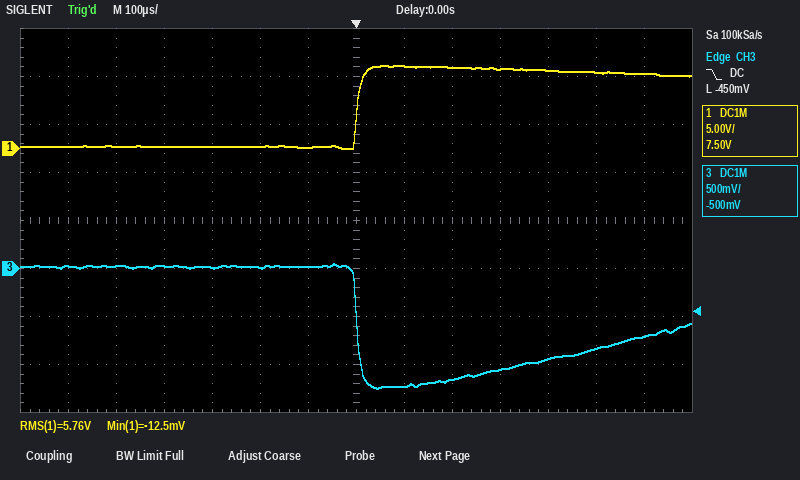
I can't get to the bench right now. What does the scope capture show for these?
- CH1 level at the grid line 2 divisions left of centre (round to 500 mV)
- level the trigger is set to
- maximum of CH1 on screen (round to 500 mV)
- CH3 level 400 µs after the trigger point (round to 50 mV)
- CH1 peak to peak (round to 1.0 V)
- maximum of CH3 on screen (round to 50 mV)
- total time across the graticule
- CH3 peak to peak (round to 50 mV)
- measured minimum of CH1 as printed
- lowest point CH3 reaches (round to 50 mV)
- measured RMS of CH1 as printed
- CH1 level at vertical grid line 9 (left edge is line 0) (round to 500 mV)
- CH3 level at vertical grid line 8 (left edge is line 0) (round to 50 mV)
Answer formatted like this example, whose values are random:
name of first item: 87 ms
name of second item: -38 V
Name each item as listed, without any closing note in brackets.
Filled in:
CH1 level at the grid line 2 divisions left of centre: 0.0 V
level the trigger is set to: -450 mV
maximum of CH1 on screen: 8.5 V
CH3 level 400 µs after the trigger point: -950 mV
CH1 peak to peak: 9.0 V
maximum of CH3 on screen: 50 mV
total time across the graticule: 1.4 ms
CH3 peak to peak: 1.30 V
measured minimum of CH1 as printed: -12.5 mV
lowest point CH3 reaches: -1.25 V
measured RMS of CH1 as printed: 5.76 V
CH1 level at vertical grid line 9 (left edge is line 0): 8.5 V
CH3 level at vertical grid line 8 (left edge is line 0): -1.25 V
